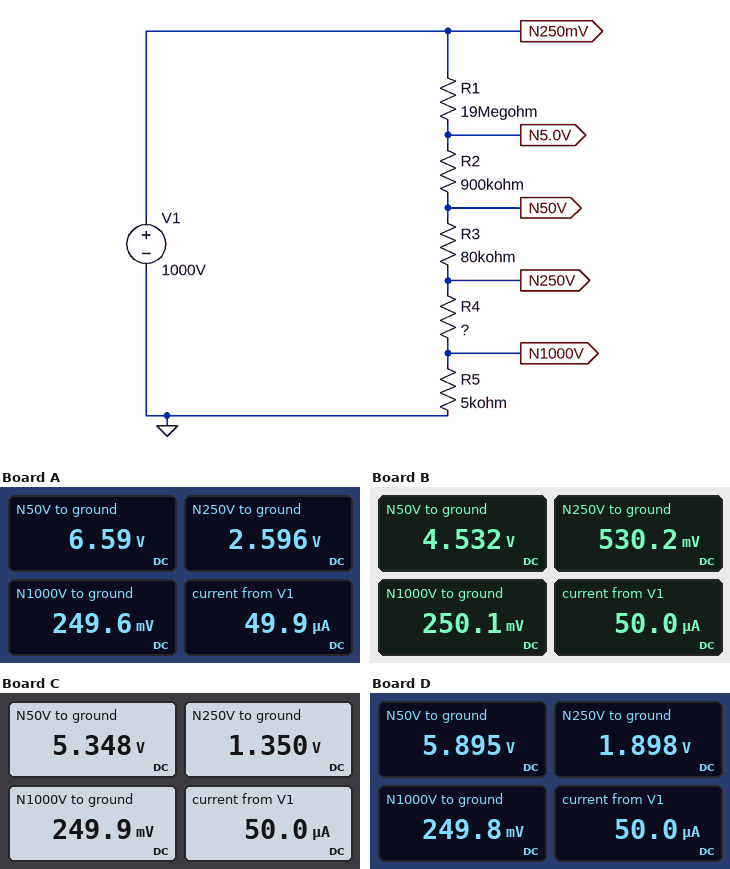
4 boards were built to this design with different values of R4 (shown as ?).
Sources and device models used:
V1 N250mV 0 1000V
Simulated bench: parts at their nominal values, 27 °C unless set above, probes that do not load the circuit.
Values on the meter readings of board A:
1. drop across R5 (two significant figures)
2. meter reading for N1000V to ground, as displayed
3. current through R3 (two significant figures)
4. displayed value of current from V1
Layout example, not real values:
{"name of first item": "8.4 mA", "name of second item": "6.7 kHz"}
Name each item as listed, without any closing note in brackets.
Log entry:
{"drop across R5": "250 mV", "meter reading for N1000V to ground, as displayed": "249.6 mV", "current through R3": "50 µA", "displayed value of current from V1": "49.9 µA"}
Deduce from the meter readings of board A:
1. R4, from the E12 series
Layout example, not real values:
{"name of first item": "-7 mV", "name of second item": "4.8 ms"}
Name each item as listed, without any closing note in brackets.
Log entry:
{"R4, from the E12 series": "47 kΩ"}
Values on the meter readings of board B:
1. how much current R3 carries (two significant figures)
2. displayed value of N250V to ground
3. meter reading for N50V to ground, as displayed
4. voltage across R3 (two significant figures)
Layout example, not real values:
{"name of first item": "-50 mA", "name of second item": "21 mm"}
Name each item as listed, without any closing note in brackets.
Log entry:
{"how much current R3 carries": "50 µA", "displayed value of N250V to ground": "530.2 mV", "meter reading for N50V to ground, as displayed": "4.532 V", "voltage across R3": "4.0 V"}
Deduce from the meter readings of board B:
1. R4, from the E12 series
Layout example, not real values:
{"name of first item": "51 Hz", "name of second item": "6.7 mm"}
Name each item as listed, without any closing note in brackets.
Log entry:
{"R4, from the E12 series": "5.6 kΩ"}
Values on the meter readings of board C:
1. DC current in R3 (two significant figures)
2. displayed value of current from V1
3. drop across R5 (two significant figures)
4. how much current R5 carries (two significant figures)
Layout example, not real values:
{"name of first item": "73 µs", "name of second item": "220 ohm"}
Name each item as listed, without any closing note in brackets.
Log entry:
{"DC current in R3": "50 µA", "displayed value of current from V1": "50.0 µA", "drop across R5": "250 mV", "how much current R5 carries": "50 µA"}
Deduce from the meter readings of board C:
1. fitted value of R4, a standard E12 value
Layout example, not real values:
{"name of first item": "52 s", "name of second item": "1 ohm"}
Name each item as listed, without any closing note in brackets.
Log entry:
{"fitted value of R4, a standard E12 value": "22 kΩ"}
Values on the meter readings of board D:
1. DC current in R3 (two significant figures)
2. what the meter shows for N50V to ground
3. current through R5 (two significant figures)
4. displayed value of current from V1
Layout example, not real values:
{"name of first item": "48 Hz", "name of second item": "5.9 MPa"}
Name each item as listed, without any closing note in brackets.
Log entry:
{"DC current in R3": "50 µA", "what the meter shows for N50V to ground": "5.895 V", "current through R5": "50 µA", "displayed value of current from V1": "50.0 µA"}
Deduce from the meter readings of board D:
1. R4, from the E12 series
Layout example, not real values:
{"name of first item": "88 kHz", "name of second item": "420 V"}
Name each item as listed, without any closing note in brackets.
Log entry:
{"R4, from the E12 series": "33 kΩ"}
